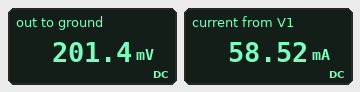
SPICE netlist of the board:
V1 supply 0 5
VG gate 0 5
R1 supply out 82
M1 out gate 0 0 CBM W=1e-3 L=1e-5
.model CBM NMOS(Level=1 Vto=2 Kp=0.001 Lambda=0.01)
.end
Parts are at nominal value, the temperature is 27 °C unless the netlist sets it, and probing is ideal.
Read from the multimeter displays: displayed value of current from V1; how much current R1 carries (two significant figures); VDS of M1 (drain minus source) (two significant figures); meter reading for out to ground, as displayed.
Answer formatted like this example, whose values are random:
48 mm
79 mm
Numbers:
58.52 mA
59 mA
200 mV
201.4 mV
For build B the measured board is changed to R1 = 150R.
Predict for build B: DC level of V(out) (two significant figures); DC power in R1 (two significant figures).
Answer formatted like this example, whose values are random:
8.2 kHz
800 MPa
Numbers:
110 mV
160 mW
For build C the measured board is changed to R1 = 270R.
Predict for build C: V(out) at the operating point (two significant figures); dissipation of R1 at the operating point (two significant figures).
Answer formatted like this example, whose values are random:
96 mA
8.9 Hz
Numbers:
62 mV
90 mW
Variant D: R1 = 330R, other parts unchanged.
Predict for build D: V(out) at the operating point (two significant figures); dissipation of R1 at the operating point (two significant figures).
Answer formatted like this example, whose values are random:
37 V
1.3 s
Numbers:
50 mV
74 mW
